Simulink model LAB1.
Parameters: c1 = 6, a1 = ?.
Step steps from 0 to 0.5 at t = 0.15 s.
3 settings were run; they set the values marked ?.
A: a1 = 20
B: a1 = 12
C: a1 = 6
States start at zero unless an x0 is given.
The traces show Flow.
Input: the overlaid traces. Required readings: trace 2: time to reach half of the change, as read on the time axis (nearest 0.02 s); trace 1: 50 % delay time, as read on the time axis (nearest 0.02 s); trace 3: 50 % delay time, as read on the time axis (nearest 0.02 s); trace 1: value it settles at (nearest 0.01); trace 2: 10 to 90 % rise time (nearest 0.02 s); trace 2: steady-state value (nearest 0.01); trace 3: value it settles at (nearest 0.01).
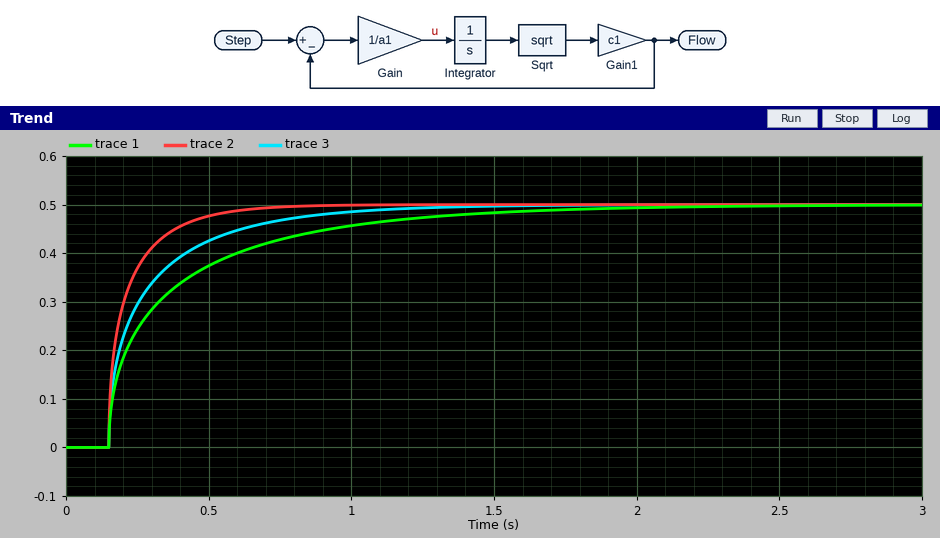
0.18 s
0.26 s
0.22 s
0.50
0.24 s
0.50
0.50
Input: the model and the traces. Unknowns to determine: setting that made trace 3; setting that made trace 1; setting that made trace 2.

B
A
C
